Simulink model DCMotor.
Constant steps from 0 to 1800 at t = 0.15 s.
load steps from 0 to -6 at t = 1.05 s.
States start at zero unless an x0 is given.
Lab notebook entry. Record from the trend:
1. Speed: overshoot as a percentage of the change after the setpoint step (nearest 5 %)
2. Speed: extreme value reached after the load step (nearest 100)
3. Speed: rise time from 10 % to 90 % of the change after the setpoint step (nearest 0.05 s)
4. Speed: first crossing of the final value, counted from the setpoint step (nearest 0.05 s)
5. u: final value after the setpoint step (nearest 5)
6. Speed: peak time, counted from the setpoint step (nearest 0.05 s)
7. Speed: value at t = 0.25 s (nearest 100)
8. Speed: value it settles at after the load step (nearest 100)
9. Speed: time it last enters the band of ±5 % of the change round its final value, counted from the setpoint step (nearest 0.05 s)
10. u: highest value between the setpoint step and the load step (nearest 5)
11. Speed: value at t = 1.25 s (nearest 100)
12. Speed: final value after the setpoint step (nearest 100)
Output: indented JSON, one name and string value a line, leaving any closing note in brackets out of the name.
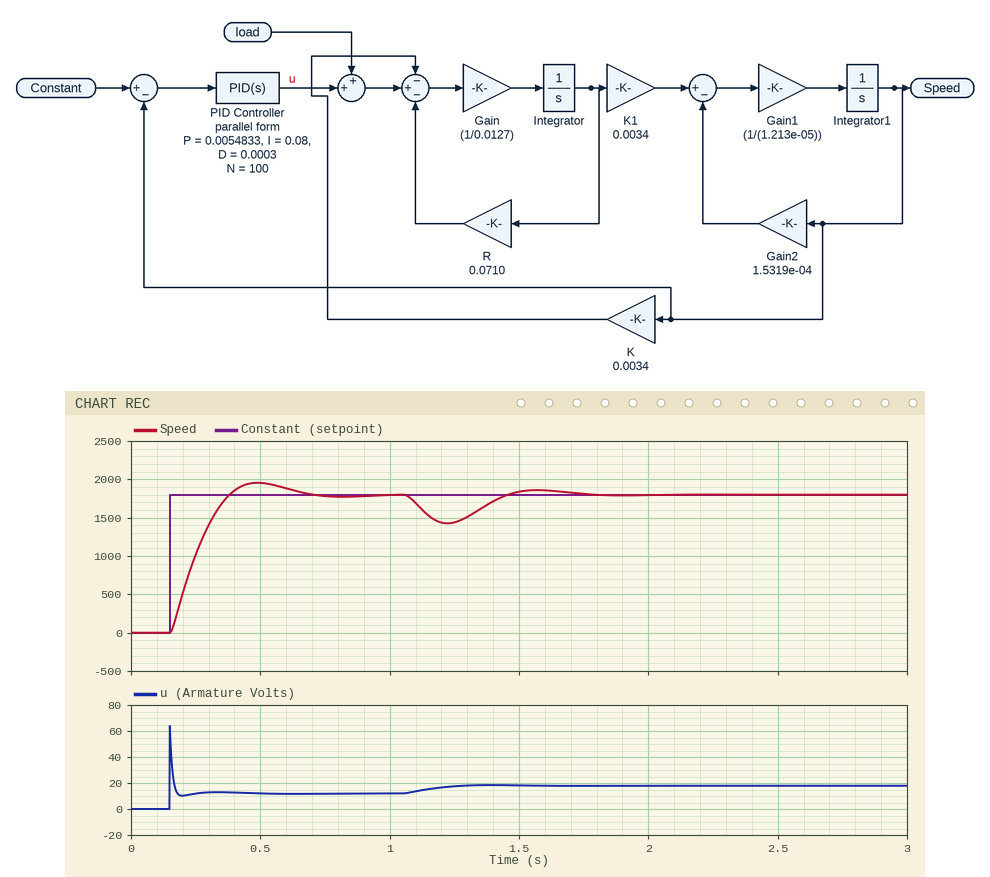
{
  "Speed: overshoot as a percentage of the change after the setpoint step": "10 %",
  "Speed: extreme value reached after the load step": "1400",
  "Speed: rise time from 10 % to 90 % of the change after the setpoint step": "0.15 s",
  "Speed: first crossing of the final value, counted from the setpoint step": "0.25 s",
  "u: final value after the setpoint step": "10",
  "Speed: peak time, counted from the setpoint step": "0.35 s",
  "Speed: value at t = 0.25 s": "1000",
  "Speed: value it settles at after the load step": "1800",
  "Speed: time it last enters the band of ±5 % of the change round its final value, counted from the setpoint step": "0.45 s",
  "u: highest value between the setpoint step and the load step": "65",
  "Speed: value at t = 1.25 s": "1400",
  "Speed: final value after the setpoint step": "1800"
}
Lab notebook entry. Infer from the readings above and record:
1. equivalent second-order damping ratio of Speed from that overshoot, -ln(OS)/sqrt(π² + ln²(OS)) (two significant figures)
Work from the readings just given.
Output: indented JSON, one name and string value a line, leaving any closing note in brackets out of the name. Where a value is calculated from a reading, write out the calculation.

{
  "equivalent second-order damping ratio of Speed from that overshoot, -ln(OS)/sqrt(π² + ln²(OS))": "ln(0.1) = -2.303; 2.303 / sqrt(9.870 + 5.302) = 0.59"
}
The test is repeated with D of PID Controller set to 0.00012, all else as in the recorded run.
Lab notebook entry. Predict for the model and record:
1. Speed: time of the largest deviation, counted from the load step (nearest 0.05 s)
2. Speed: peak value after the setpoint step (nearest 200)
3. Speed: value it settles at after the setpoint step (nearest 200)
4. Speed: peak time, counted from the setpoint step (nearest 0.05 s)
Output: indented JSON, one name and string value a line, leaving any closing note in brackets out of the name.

{
  "Speed: time of the largest deviation, counted from the load step": "0.15 s",
  "Speed: peak value after the setpoint step": "2000",
  "Speed: value it settles at after the setpoint step": "1800",
  "Speed: peak time, counted from the setpoint step": "0.30 s"
}
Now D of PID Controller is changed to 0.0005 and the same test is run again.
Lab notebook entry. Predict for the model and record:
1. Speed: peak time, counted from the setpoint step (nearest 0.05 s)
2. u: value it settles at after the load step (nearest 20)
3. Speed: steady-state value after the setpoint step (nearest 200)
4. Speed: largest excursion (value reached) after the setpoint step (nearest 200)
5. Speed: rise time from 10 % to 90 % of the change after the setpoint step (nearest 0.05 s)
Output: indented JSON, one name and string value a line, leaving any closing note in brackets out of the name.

{
  "Speed: peak time, counted from the setpoint step": "0.40 s",
  "u: value it settles at after the load step": "20",
  "Speed: steady-state value after the setpoint step": "1800",
  "Speed: largest excursion (value reached) after the setpoint step": "2000",
  "Speed: rise time from 10 % to 90 % of the change after the setpoint step": "0.20 s"
}
